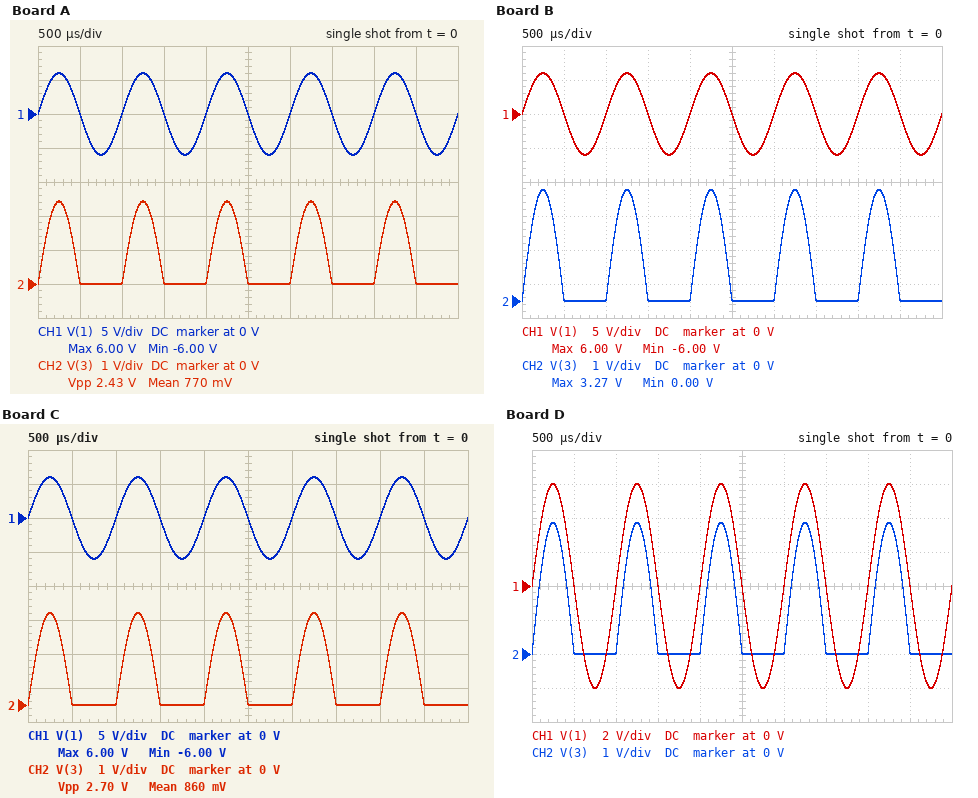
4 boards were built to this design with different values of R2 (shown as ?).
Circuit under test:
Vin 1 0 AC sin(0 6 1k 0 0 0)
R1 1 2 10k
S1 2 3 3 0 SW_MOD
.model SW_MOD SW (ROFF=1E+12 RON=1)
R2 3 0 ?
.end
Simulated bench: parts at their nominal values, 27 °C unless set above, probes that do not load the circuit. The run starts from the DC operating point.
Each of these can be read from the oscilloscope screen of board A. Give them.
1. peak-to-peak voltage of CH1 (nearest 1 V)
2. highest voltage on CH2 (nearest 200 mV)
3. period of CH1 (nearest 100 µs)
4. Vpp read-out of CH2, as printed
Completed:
12 V
2.4 V
1.0 ms
2.43 V
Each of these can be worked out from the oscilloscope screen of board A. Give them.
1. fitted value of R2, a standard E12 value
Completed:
6.8 kΩ
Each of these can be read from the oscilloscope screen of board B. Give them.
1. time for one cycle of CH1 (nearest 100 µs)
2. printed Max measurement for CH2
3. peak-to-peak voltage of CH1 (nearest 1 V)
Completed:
1.0 ms
3.27 V
12 V
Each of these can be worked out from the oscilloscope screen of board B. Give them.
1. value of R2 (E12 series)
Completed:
12 kΩ
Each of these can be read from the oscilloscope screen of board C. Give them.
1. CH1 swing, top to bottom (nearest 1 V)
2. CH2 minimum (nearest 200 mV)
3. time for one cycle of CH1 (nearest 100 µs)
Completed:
12 V
0 V
1.0 ms
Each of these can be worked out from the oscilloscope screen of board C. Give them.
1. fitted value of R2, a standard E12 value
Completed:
8.2 kΩ
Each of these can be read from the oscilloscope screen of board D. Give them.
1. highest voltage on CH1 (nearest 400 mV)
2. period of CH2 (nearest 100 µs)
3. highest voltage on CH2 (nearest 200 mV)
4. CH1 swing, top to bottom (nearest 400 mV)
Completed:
6.0 V
1.0 ms
3.8 V
12.0 V
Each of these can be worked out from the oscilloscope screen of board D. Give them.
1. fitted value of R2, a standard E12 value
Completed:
18 kΩ
